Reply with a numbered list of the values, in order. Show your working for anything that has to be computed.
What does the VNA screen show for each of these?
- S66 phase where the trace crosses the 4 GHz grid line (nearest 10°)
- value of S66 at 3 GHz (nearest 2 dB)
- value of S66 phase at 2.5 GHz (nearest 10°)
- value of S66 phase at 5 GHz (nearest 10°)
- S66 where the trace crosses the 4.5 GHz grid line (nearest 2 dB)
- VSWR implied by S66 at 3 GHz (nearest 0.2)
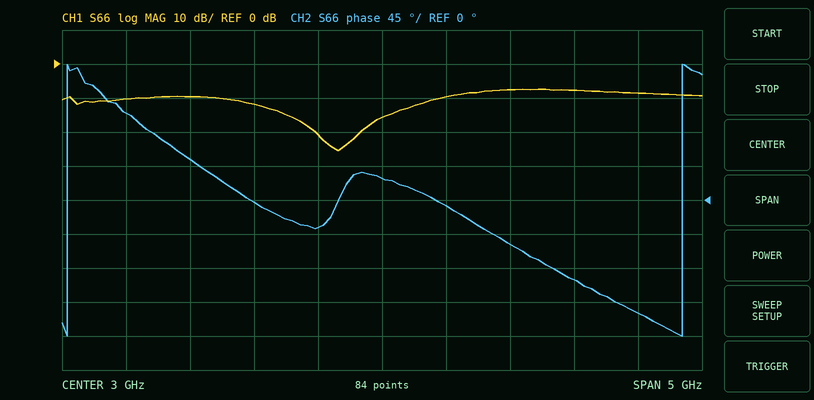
1. -60°
2. -16 dB
3. -40°
4. -150°
5. -8 dB
6. |Γ| = 10^(-16/20) = 0.1585; VSWR = (1 + 0.1585)/(1 − 0.1585) ≈ 1.4
